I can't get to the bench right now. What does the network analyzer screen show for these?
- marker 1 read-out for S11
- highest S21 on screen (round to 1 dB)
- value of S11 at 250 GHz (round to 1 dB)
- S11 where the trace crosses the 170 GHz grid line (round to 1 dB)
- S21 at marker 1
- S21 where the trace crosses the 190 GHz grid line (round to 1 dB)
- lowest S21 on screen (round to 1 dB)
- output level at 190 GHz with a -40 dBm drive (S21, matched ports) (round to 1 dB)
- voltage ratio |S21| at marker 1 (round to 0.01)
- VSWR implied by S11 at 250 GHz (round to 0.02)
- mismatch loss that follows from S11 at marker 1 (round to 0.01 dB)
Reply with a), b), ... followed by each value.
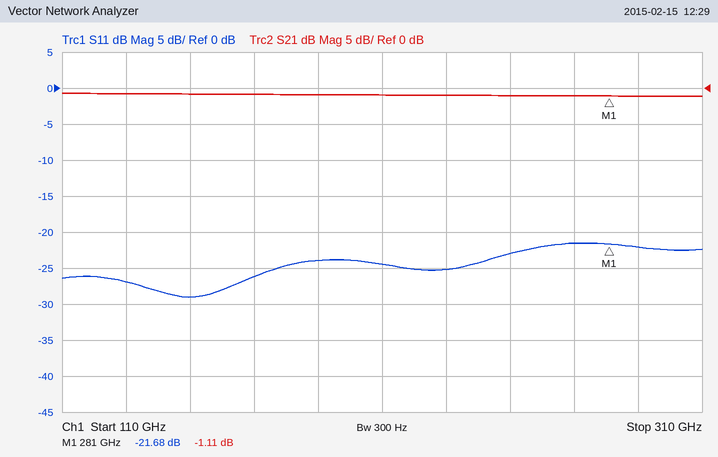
a) -21.68 dB
b) -1 dB
c) -23 dB
d) -26 dB
e) -1.11 dB
f) -1 dB
g) -1 dB
h) -41 dBm
i) 0.88
j) 1.16
k) 0.03 dB
